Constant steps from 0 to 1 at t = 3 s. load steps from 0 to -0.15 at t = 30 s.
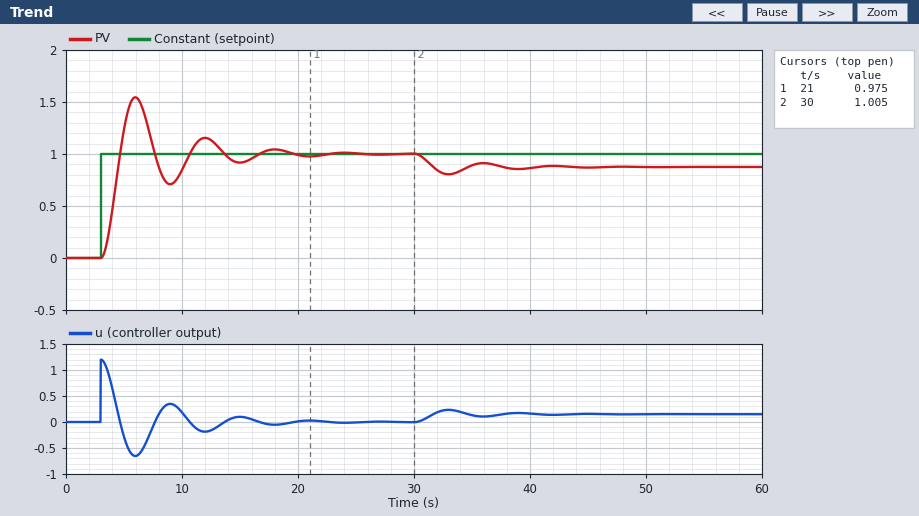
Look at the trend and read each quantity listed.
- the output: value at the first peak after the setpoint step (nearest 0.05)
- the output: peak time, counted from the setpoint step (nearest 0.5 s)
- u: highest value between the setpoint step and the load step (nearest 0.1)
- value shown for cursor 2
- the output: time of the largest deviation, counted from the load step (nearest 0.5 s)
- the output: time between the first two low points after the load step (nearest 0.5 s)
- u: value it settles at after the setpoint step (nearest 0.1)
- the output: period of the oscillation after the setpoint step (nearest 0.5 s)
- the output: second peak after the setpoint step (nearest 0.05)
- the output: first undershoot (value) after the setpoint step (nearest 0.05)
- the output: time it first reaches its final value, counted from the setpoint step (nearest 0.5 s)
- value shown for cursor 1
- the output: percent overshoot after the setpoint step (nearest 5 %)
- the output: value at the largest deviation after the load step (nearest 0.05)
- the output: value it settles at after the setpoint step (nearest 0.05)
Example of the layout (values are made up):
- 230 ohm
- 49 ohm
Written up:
- 1.55
- 3.0 s
- 1.2
- 1.005
- 3.0 s
- 6.0 s
- 0.0
- 6.0 s
- 1.15
- 0.70
- 1.5 s
- 0.975
- 55 %
- 0.80
- 1.00
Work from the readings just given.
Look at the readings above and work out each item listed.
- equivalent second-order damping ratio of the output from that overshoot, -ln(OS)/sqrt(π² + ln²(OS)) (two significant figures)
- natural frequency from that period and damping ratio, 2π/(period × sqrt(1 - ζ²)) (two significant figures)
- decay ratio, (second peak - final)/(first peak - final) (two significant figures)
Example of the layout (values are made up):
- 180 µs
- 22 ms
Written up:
- 0.19
- 1.1 rad/s
- 0.27
